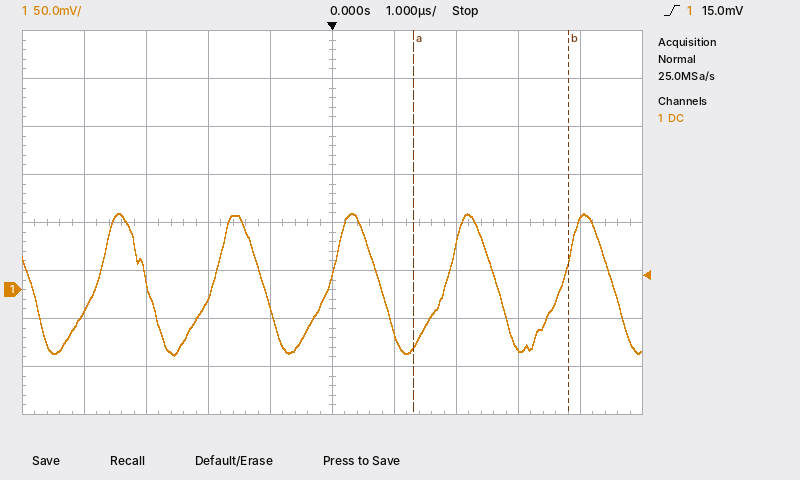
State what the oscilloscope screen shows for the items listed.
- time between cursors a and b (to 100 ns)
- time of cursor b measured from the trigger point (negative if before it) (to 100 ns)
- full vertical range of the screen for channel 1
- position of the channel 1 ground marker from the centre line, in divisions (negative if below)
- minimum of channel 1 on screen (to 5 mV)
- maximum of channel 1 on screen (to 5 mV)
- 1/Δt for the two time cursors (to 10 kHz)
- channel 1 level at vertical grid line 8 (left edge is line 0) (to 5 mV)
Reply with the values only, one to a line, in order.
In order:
2.5 µs
+3.8 µs
400 mV
-1.4 div
-70 mV
80 mV
400 kHz
-60 mV
